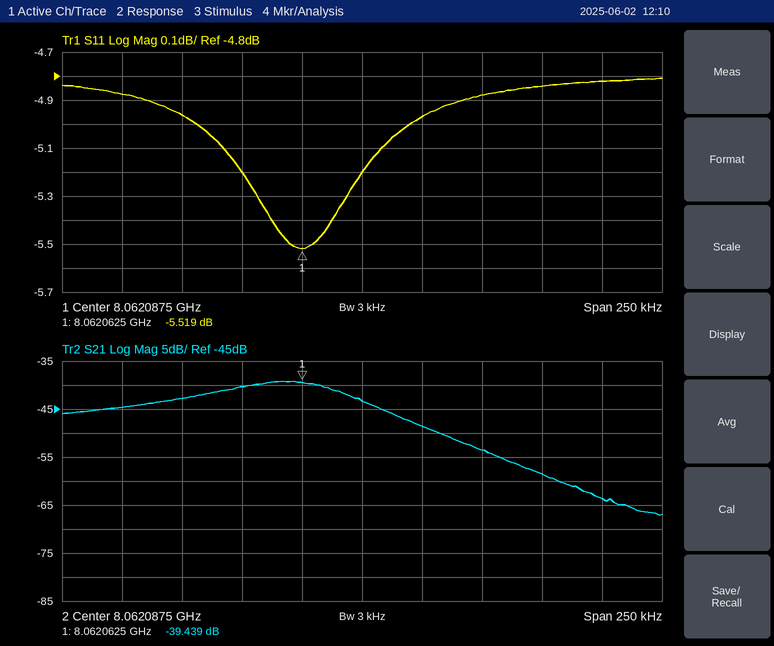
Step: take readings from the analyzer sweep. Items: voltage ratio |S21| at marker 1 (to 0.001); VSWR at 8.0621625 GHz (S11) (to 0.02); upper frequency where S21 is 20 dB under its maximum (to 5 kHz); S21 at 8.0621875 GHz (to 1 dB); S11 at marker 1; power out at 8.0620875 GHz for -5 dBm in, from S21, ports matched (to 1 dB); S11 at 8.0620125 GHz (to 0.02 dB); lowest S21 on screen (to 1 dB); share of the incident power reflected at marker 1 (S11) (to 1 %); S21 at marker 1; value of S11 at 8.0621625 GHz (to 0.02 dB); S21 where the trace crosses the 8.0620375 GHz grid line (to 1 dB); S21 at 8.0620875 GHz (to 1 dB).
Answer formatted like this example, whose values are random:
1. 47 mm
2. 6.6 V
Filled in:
1. 0.011
2. 3.68
3. 8.062165 GHz
4. -64 dB
5. -5.519 dB
6. -48 dBm
7. -4.96 dB
8. -67 dB
9. 28 %
10. -39.439 dB
11. -4.84 dB
12. -40 dB
13. -43 dB
